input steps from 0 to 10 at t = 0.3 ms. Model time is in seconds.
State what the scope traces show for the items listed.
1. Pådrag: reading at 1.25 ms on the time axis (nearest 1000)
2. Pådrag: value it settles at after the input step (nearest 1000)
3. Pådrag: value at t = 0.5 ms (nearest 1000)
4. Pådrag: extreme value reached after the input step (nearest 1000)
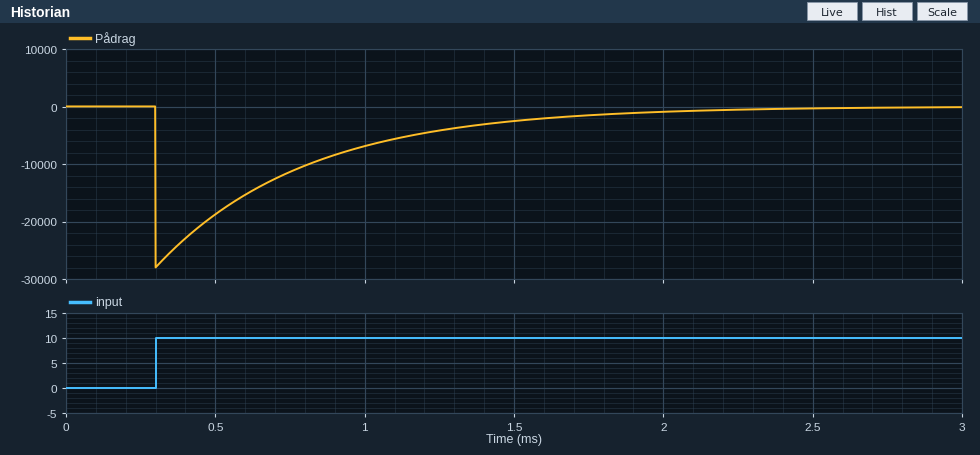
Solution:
-4000
0
-19000
-28000
